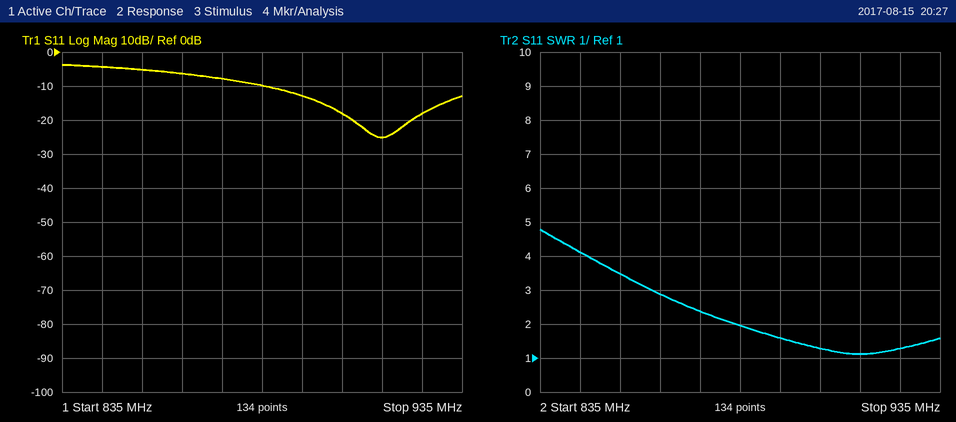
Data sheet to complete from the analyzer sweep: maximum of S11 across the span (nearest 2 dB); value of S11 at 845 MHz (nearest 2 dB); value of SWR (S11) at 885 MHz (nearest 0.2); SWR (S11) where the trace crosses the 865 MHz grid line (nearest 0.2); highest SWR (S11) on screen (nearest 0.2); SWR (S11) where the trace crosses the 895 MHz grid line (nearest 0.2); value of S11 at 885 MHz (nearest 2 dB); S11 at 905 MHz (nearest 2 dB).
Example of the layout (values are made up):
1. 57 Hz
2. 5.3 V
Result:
1. -4 dB
2. -4 dB
3. 2.0
4. 2.8
5. 4.8
6. 1.6
7. -10 dB
8. -18 dB
